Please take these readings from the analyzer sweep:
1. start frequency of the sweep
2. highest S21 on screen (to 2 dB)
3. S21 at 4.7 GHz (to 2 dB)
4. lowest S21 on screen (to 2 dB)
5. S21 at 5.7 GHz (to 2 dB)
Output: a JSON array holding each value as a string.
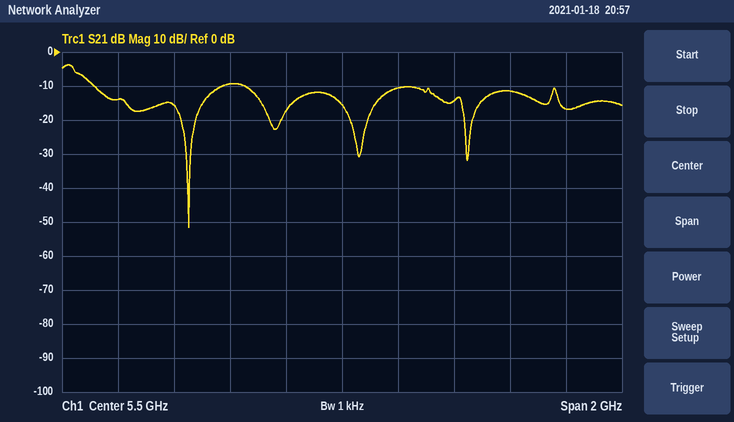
["4.5 GHz", "-4 dB", "-14 dB", "-52 dB", "-10 dB"]
